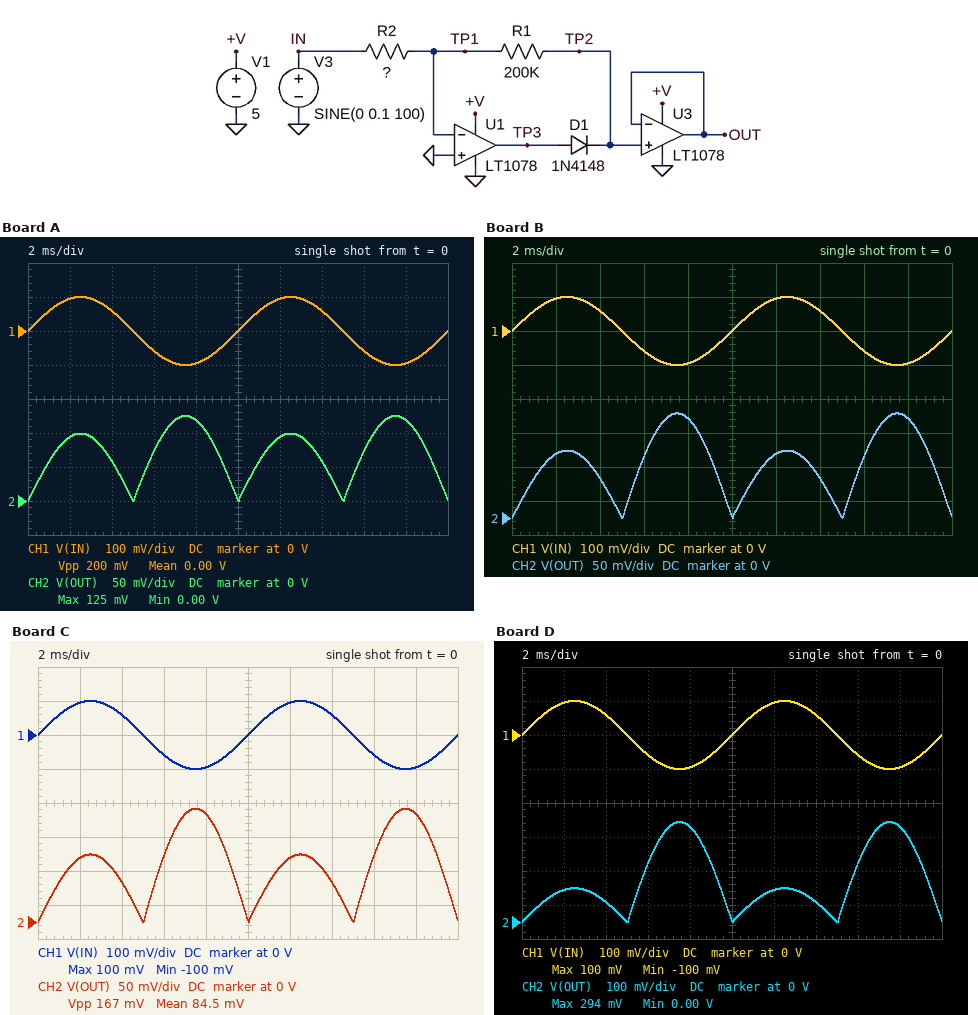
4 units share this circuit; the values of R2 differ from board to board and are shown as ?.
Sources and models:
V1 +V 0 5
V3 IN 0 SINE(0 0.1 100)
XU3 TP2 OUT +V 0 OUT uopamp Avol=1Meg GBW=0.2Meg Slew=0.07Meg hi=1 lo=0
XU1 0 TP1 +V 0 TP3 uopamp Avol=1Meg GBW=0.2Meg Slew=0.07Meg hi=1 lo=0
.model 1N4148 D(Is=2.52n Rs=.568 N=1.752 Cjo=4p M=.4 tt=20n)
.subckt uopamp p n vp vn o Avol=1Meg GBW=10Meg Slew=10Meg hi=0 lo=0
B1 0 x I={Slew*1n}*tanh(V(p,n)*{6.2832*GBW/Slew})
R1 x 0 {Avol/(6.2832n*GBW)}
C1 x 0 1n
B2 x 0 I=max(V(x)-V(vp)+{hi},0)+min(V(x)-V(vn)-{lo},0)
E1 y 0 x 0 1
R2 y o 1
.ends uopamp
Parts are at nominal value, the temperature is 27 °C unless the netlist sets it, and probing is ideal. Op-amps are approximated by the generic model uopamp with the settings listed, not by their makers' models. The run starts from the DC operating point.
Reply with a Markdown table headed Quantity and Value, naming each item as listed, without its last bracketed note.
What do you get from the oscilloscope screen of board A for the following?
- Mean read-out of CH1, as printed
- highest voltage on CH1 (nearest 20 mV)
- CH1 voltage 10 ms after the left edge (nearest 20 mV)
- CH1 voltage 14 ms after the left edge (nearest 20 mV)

| Quantity | Value |
|---|---|
| Mean read-out of CH1, as printed | 0.00 V |
| highest voltage on CH1 | 100 mV |
| CH1 voltage 10 ms after the left edge | 0 V |
| CH1 voltage 14 ms after the left edge | 60 mV |
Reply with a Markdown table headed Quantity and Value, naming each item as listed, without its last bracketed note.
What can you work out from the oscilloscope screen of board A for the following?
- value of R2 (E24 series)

| Quantity | Value |
|---|---|
| value of R2 | 160 kΩ |
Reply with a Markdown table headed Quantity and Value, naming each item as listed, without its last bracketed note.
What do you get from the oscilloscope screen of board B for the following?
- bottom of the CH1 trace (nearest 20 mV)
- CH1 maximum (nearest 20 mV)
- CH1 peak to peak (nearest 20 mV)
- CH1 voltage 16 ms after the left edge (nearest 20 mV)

| Quantity | Value |
|---|---|
| bottom of the CH1 trace | -100 mV |
| CH1 maximum | 100 mV |
| CH1 peak to peak | 200 mV |
| CH1 voltage 16 ms after the left edge | -60 mV |
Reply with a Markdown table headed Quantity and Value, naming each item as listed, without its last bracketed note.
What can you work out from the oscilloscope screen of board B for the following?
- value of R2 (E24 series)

| Quantity | Value |
|---|---|
| value of R2 | 130 kΩ |
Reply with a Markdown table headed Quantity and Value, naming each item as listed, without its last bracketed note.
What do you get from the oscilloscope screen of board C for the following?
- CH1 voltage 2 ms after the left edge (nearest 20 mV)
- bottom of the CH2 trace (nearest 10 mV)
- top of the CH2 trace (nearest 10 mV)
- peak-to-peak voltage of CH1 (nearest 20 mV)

| Quantity | Value |
|---|---|
| CH1 voltage 2 ms after the left edge | 100 mV |
| bottom of the CH2 trace | 0 V |
| top of the CH2 trace | 170 mV |
| peak-to-peak voltage of CH1 | 200 mV |
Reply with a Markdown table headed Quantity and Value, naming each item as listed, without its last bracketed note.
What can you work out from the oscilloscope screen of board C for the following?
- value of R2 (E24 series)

| Quantity | Value |
|---|---|
| value of R2 | 120 kΩ |
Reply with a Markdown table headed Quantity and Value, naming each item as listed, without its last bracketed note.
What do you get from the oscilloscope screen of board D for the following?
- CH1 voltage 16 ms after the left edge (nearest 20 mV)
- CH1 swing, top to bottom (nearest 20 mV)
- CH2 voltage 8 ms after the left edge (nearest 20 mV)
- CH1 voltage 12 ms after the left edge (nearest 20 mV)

| Quantity | Value |
|---|---|
| CH1 voltage 16 ms after the left edge | -60 mV |
| CH1 swing, top to bottom | 200 mV |
| CH2 voltage 8 ms after the left edge | 280 mV |
| CH1 voltage 12 ms after the left edge | 100 mV |
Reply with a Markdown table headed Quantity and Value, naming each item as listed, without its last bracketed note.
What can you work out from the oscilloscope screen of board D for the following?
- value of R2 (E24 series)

| Quantity | Value |
|---|---|
| value of R2 | 68 kΩ |
